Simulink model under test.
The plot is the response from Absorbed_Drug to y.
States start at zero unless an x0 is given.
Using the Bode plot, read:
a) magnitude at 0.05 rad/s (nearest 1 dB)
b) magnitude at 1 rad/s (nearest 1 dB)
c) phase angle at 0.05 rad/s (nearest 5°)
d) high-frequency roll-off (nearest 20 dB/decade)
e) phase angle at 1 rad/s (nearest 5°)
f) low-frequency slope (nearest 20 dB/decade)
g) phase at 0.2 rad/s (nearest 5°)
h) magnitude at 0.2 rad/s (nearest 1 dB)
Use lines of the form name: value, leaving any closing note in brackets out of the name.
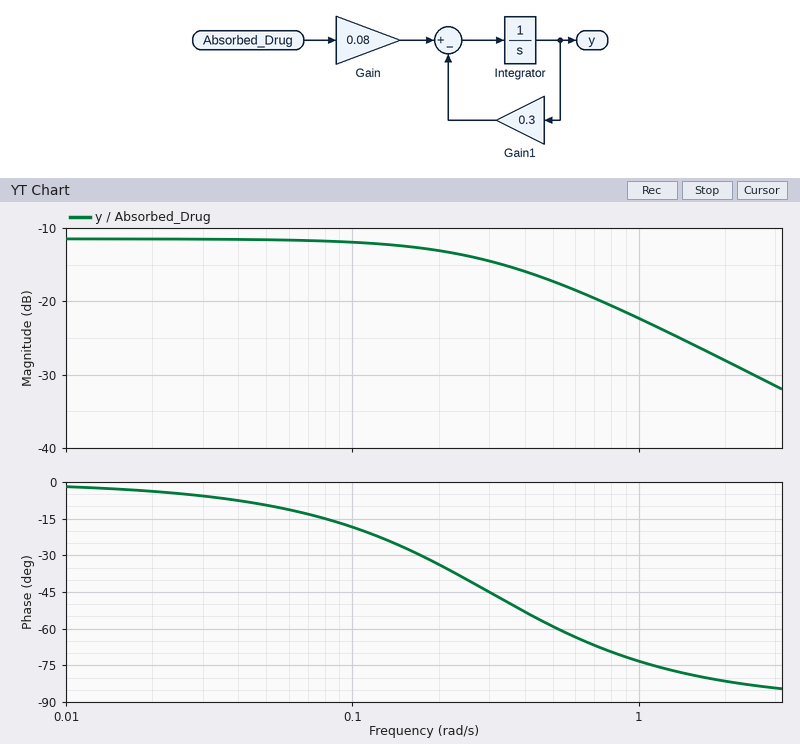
magnitude at 0.05 rad/s: -12 dB
magnitude at 1 rad/s: -22 dB
phase angle at 0.05 rad/s: -10°
high-frequency roll-off: -20 dB/decade
phase angle at 1 rad/s: -75°
low-frequency slope: 0 dB/decade
phase at 0.2 rad/s: -35°
magnitude at 0.2 rad/s: -13 dB
